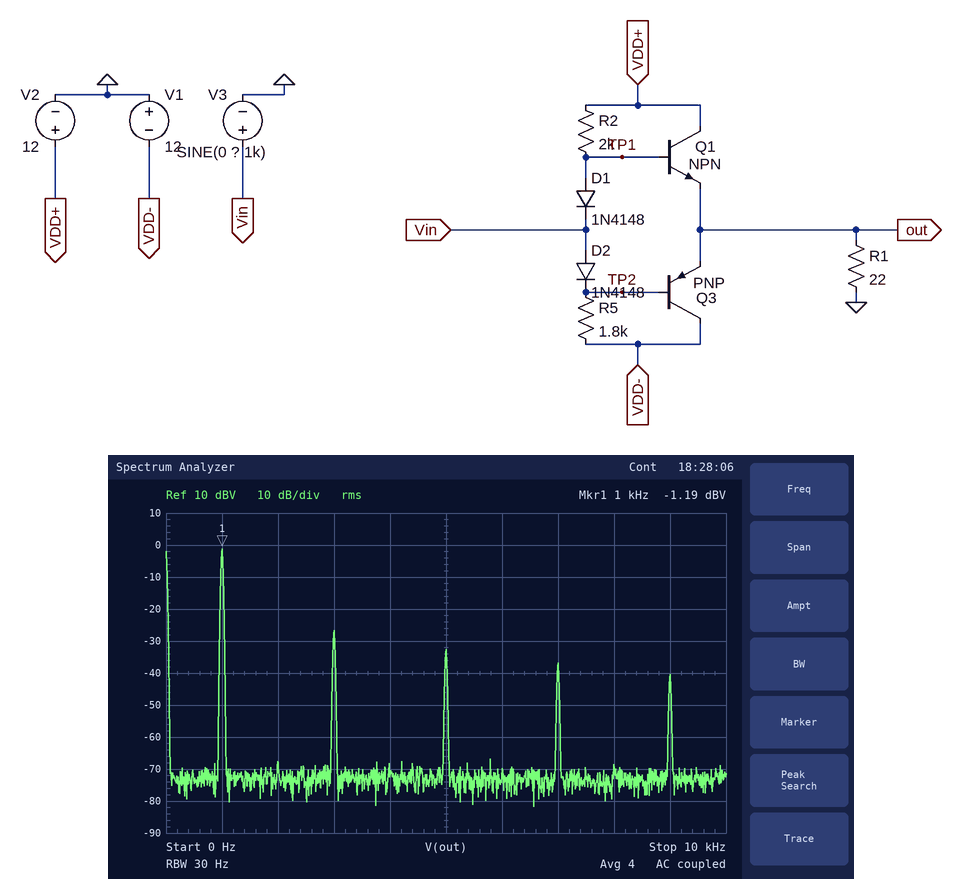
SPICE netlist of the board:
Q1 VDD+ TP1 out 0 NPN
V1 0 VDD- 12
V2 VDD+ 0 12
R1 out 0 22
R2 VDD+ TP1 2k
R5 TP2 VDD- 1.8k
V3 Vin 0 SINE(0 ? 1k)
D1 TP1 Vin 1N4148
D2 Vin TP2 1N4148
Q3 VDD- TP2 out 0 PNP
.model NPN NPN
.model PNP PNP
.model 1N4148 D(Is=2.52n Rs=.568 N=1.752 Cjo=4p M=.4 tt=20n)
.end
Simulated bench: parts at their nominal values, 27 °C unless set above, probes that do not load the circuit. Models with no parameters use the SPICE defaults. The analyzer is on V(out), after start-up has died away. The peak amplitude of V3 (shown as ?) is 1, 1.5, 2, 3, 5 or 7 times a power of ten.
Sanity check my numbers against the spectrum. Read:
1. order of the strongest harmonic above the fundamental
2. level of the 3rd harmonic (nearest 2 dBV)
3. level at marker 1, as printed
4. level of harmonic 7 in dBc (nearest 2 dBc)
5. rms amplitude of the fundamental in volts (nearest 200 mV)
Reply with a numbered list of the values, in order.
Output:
1. 3
2. -26 dBV
3. -1.19 dBV
4. -36 dBc
5. 800 mV
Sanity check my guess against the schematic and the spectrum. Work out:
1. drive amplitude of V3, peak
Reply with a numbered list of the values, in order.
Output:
1. 1.5 V
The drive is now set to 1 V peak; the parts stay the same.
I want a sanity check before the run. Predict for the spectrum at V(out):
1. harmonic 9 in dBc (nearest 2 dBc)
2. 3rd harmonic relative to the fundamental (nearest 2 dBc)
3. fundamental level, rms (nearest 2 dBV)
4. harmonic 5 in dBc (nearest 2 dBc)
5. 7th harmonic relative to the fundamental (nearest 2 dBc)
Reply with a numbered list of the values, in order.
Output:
1. -38 dBc
2. -22 dBc
3. -6 dBV
4. -28 dBc
5. -34 dBc
